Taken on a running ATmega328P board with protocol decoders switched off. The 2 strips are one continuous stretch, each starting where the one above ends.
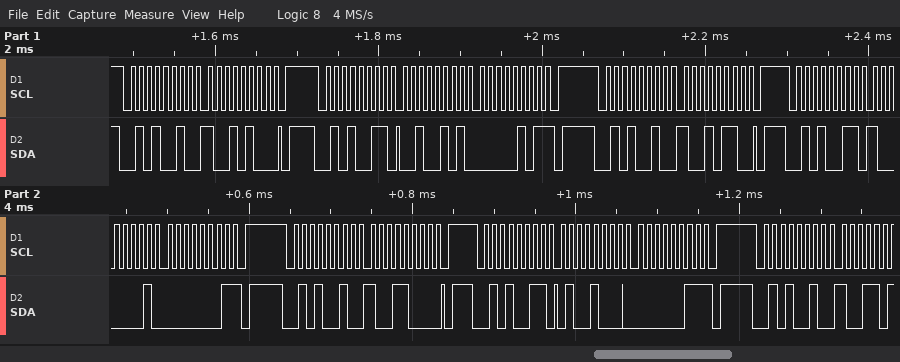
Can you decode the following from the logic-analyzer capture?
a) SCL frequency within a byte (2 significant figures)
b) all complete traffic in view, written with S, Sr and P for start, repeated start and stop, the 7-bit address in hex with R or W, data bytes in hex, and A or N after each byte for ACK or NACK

100 kHz
S 29W A 94 A P S 29R A 25 A 05 N P S 29W A 96 A P S 29R A 81 A 01 N P S 29W A 98 A P S 29R A 48 A 03 N P S 29W A
